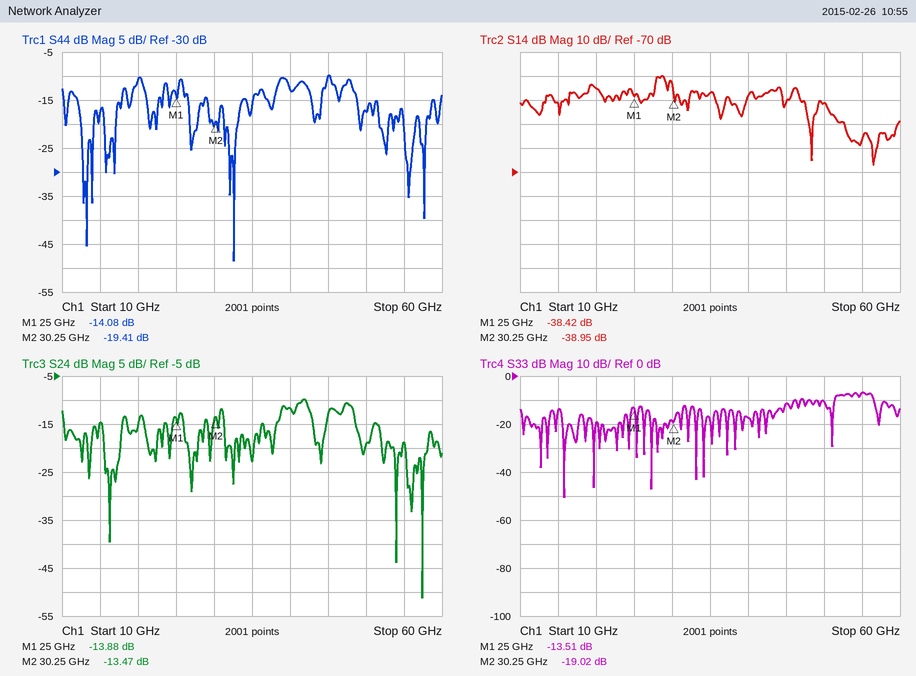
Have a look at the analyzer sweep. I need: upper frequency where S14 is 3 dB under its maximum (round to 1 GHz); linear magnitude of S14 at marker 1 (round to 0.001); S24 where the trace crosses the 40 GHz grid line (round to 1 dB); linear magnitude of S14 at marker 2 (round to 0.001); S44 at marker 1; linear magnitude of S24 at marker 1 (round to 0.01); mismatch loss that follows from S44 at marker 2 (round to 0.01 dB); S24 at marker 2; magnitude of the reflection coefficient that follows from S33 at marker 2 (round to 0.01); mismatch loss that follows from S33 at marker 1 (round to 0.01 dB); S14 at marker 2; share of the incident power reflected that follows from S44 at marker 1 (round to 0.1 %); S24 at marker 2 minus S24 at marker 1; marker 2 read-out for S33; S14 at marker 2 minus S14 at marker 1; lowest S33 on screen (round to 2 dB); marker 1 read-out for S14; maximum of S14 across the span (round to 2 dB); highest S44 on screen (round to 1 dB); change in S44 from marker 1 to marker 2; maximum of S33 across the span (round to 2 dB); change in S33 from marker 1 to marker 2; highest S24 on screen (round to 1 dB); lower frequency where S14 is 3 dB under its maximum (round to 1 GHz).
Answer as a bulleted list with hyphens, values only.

- 29 GHz
- 0.012
- -12 dB
- 0.011
- -14.08 dB
- 0.20
- 0.05 dB
- -13.47 dB
- 0.11
- 0.20 dB
- -38.95 dB
- 3.9 %
- 0.41 dB
- -19.02 dB
- -0.53 dB
- -50 dB
- -38.42 dB
- -30 dB
- -10 dB
- -5.33 dB
- -6 dB
- -5.51 dB
- -10 dB
- 28 GHz
